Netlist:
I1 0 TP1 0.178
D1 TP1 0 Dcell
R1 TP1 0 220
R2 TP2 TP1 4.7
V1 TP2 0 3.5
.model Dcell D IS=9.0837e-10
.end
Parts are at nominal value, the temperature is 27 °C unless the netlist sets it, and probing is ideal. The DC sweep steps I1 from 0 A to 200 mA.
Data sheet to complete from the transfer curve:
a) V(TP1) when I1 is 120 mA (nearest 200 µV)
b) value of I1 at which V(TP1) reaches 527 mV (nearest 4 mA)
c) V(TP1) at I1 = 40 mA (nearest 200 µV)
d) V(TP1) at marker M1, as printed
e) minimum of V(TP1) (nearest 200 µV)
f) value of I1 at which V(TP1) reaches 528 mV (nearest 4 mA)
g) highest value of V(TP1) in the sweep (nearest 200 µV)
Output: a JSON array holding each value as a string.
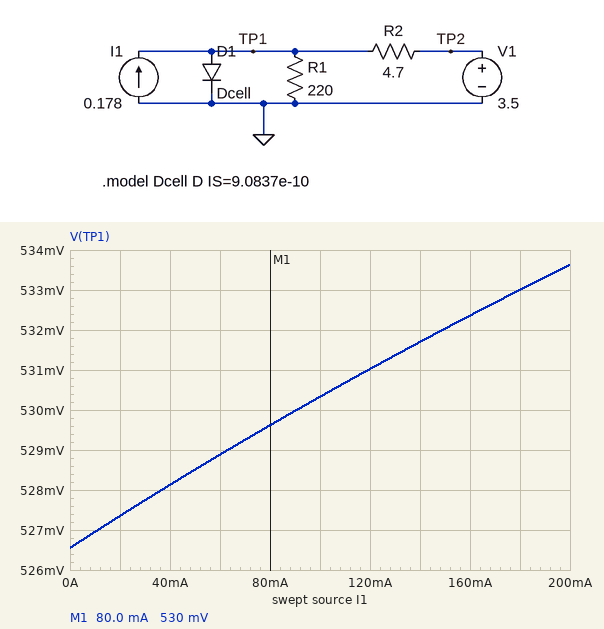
["531.0 mV", "12 mA", "528.2 mV", "530 mV", "526.6 mV", "36 mA", "533.6 mV"]
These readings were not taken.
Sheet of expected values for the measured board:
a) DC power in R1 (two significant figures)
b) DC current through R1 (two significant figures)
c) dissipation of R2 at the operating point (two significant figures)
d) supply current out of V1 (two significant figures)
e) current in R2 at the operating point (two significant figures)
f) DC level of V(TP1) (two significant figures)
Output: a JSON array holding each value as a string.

["1.3 mW", "2.4 mA", "1.9 W", "630 mA", "630 mA", "530 mV"]
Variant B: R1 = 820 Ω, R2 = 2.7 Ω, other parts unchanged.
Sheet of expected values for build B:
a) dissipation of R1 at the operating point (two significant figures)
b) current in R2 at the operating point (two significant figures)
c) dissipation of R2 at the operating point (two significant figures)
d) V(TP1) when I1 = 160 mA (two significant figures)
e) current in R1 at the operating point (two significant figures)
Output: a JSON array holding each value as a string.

["360 µW", "1.1 A", "3.2 W", "540 mV", "660 µA"]
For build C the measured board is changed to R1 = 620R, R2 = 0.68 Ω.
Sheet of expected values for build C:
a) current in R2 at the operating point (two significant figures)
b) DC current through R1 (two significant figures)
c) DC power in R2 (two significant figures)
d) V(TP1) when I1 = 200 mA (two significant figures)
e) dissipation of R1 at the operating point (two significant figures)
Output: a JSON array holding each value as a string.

["4.3 A", "930 µA", "13 W", "580 mV", "540 µW"]
